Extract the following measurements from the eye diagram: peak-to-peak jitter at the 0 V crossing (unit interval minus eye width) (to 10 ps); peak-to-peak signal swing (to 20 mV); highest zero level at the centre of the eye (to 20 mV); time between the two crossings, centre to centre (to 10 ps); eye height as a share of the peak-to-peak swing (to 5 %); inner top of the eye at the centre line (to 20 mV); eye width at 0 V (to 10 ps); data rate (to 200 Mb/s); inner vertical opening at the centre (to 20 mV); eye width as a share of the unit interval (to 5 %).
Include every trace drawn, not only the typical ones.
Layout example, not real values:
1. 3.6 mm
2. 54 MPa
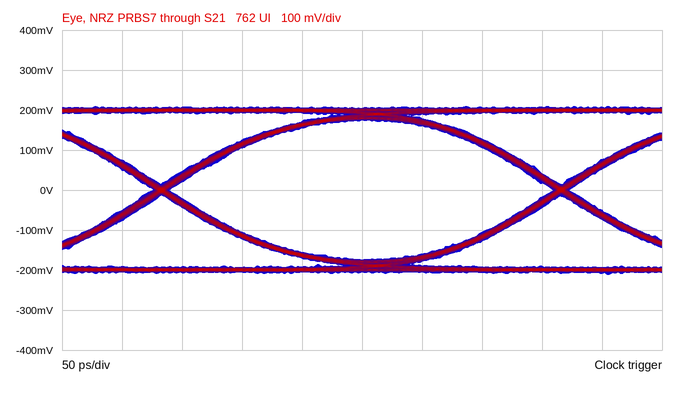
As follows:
1. 10 ps
2. 420 mV
3. -180 mV
4. 330 ps
5. 85 %
6. 180 mV
7. 320 ps
8. 3.0 Gb/s
9. 360 mV
10. 95 %
